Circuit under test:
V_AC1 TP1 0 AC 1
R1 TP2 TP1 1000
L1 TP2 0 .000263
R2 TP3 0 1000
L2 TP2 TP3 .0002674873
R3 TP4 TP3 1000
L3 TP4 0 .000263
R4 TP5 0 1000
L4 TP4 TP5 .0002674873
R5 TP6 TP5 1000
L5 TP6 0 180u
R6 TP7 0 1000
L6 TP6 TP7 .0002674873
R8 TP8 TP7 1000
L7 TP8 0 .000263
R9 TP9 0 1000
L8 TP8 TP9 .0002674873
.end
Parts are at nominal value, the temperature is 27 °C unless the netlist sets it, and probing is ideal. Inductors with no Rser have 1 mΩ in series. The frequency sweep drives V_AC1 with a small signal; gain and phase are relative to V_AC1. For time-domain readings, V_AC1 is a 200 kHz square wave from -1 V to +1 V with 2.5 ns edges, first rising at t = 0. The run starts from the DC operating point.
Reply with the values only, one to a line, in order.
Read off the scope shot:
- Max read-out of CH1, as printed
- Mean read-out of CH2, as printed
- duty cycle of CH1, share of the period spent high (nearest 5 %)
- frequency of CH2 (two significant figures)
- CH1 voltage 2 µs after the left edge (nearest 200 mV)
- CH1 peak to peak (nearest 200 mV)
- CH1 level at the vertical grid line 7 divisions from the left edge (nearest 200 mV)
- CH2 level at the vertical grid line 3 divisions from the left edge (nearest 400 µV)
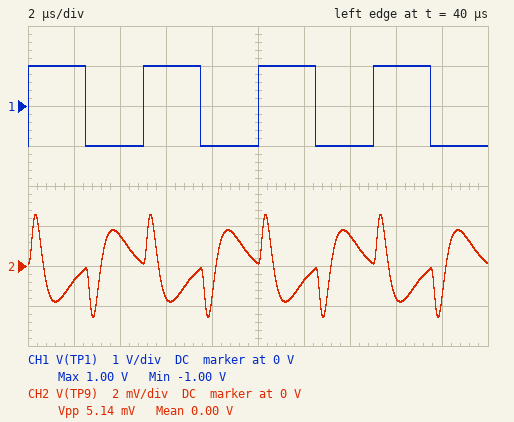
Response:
1.00 V
0.00 V
50 %
200 kHz
1.0 V
2.0 V
-1.0 V
-1.6 mV
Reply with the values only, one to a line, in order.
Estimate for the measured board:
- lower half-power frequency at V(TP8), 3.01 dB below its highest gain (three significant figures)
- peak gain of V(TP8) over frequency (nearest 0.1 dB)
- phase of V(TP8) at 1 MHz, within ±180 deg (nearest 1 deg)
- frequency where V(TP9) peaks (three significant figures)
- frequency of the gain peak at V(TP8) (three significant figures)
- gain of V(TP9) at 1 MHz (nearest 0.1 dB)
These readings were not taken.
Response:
476 kHz
-47.2 dB
5 deg
622 kHz
1.18 MHz
-53.2 dB
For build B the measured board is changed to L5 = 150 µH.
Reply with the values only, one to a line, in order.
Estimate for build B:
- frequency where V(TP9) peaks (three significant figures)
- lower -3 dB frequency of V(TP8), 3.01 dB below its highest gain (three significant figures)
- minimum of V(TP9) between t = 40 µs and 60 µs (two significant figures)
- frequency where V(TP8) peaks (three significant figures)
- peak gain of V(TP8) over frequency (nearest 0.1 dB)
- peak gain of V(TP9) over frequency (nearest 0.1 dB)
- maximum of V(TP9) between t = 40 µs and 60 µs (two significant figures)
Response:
633 kHz
489 kHz
-2.3 mV
1.21 MHz
-48.0 dB
-52.9 dB
2.3 mV
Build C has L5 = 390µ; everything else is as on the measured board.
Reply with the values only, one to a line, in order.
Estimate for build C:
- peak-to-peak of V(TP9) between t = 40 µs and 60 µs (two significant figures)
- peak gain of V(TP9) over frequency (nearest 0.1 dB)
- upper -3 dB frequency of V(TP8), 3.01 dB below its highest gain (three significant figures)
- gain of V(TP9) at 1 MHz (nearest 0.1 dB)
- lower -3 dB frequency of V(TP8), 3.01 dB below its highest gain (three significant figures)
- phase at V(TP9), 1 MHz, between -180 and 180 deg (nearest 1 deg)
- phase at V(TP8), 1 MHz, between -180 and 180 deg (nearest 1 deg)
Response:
7.7 mV
-49.1 dB
2.22 MHz
-50.6 dB
423 kHz
-65 deg
-5 deg
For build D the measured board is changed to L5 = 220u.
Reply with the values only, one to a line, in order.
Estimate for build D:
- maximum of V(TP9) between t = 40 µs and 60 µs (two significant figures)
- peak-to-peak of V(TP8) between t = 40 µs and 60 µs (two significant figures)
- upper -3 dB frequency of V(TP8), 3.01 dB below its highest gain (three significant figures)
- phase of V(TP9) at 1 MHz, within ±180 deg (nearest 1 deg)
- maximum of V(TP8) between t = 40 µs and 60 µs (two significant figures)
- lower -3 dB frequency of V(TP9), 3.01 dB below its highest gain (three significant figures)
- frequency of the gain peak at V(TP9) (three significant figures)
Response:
2.9 mV
11 mV
2.38 MHz
-57 deg
5.7 mV
288 kHz
610 kHz
